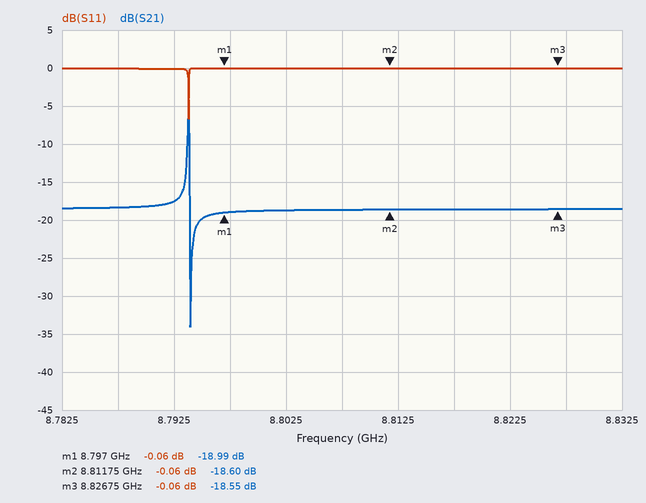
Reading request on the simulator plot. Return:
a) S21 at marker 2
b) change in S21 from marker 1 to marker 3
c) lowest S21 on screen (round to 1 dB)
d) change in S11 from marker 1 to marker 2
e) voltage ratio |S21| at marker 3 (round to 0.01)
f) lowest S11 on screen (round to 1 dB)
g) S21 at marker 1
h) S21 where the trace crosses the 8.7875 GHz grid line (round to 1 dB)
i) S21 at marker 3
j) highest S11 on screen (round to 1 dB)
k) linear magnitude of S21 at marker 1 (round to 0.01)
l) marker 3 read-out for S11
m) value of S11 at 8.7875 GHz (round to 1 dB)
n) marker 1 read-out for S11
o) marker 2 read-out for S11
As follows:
-18.60 dB
0.44 dB
-34 dB
0.00 dB
0.12
-7 dB
-18.99 dB
-18 dB
-18.55 dB
0 dB
0.11
-0.06 dB
0 dB
-0.06 dB
-0.06 dB
